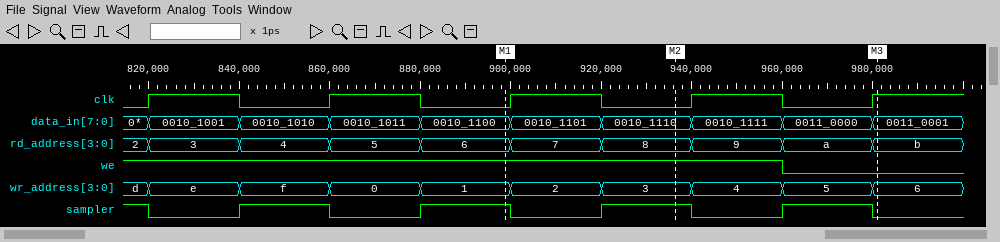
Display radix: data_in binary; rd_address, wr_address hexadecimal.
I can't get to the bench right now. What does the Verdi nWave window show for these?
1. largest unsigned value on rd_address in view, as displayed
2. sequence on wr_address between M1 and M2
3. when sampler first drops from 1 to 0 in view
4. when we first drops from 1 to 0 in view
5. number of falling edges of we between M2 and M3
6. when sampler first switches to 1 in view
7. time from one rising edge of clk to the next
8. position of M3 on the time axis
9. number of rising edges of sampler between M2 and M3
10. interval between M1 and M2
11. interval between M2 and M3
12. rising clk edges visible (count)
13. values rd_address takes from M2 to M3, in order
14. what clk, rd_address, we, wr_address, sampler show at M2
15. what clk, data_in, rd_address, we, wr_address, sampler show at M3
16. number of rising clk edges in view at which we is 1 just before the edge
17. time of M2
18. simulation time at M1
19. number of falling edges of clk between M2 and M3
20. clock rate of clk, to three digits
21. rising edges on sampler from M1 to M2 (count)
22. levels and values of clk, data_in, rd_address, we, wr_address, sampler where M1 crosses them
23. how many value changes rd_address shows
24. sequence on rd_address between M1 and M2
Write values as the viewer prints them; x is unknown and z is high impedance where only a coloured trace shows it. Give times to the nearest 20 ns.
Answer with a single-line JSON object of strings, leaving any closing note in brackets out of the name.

{"largest unsigned value on rd_address in view, as displayed": "b", "sequence on wr_address between M1 and M2": "1, 2, 3", "when sampler first drops from 1 to 0 in view": "820 ns", "when we first drops from 1 to 0 in view": "960 ns", "number of falling edges of we between M2 and M3": "1", "when sampler first switches to 1 in view": "840 ns", "time from one rising edge of clk to the next": "40 ns", "position of M3 on the time axis": "980 ns", "number of rising edges of sampler between M2 and M3": "1", "interval between M1 and M2": "40 ns", "interval between M2 and M3": "40 ns", "rising clk edges visible": "5", "values rd_address takes from M2 to M3, in order": "8, 9, a, b", "what clk, rd_address, we, wr_address, sampler show at M2": "clk=0, rd_address=8, we=1, wr_address=3, sampler=1", "what clk, data_in, rd_address, we, wr_address, sampler show at M3": "clk=1, data_in=0011_0001, rd_address=b, we=0, wr_address=6, sampler=0", "number of rising clk edges in view at which we is 1 just before the edge": "4", "time of M2": "940 ns", "simulation time at M1": "900 ns", "number of falling edges of clk between M2 and M3": "1", "clock rate of clk, to three digits": "25.0 MHz", "rising edges on sampler from M1 to M2": "1", "levels and values of clk, data_in, rd_address, we, wr_address, sampler where M1 crosses them": "clk=0, data_in=0010_1100, rd_address=6, we=1, wr_address=1, sampler=1", "how many value changes rd_address shows": "9", "sequence on rd_address between M1 and M2": "6, 7, 8"}
